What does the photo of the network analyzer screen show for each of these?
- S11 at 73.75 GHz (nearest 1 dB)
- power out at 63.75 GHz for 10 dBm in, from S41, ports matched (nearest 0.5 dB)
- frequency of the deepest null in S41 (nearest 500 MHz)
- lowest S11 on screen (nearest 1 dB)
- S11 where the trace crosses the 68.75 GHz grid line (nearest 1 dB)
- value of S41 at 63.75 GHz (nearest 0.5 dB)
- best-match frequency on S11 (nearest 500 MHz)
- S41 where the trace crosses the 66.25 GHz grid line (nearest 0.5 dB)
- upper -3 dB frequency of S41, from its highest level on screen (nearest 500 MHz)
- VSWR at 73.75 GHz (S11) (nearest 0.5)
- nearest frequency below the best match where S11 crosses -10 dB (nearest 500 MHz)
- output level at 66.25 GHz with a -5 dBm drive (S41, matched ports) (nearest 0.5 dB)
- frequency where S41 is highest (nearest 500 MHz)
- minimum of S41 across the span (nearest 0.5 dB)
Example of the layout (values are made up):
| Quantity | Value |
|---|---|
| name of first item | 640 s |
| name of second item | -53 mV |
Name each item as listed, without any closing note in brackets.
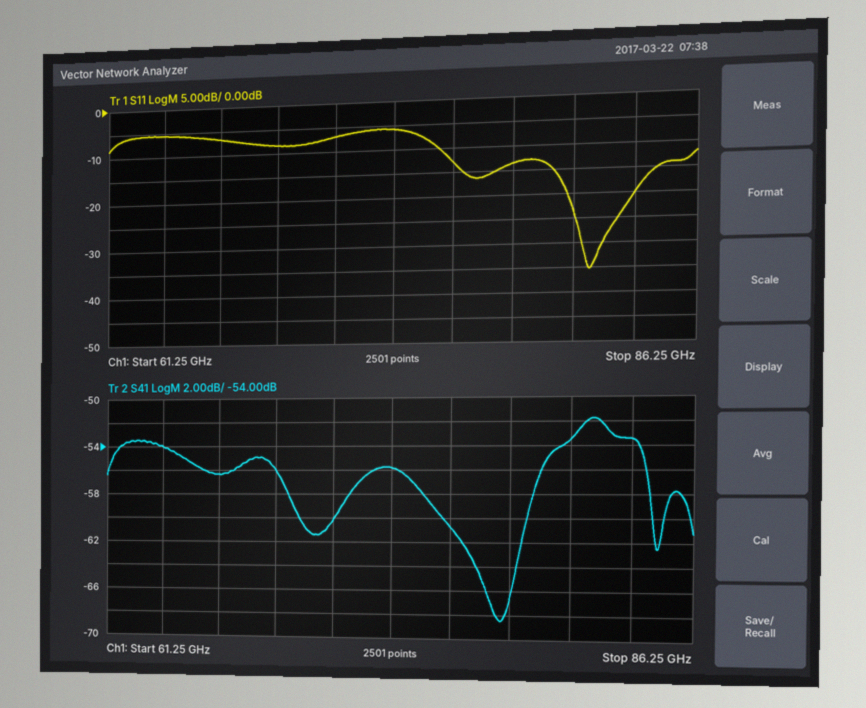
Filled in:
| Quantity | Value |
|---|---|
| S11 at 73.75 GHz | -6 dB |
| power out at 63.75 GHz for 10 dBm in, from S41, ports matched | -44.0 dBm |
| frequency of the deepest null in S41 | 78.5 GHz |
| lowest S11 on screen | -35 dB |
| S11 where the trace crosses the 68.75 GHz grid line | -8 dB |
| value of S41 at 63.75 GHz | -54.0 dB |
| best-match frequency on S11 | 82.0 GHz |
| S41 where the trace crosses the 66.25 GHz grid line | -56.5 dB |
| upper -3 dB frequency of S41, from its highest level on screen | 84.0 GHz |
| VSWR at 73.75 GHz (S11) | 3.0 |
| nearest frequency below the best match where S11 crosses -10 dB | 75.5 GHz |
| output level at 66.25 GHz with a -5 dBm drive (S41, matched ports) | -61.5 dBm |
| frequency where S41 is highest | 82.0 GHz |
| minimum of S41 across the span | -68.5 dB |
